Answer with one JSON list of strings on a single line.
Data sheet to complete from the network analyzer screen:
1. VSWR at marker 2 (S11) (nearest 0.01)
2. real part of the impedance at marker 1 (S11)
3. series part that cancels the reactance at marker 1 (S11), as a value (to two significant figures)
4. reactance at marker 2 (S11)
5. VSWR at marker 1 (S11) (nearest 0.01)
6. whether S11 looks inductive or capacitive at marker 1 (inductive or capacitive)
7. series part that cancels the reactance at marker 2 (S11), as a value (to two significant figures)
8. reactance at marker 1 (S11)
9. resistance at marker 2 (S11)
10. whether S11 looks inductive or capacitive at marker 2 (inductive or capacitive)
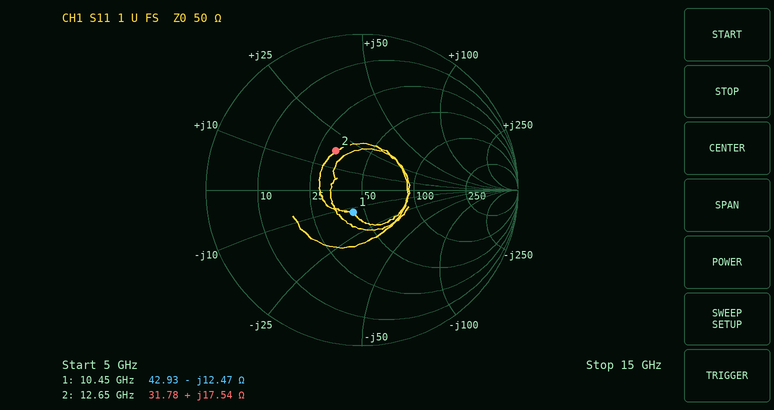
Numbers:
["1.87", "42.93 Ω", "190 pH", "+17.54 Ω", "1.36", "capacitive", "720 fF", "-12.47 Ω", "31.78 Ω", "inductive"]
